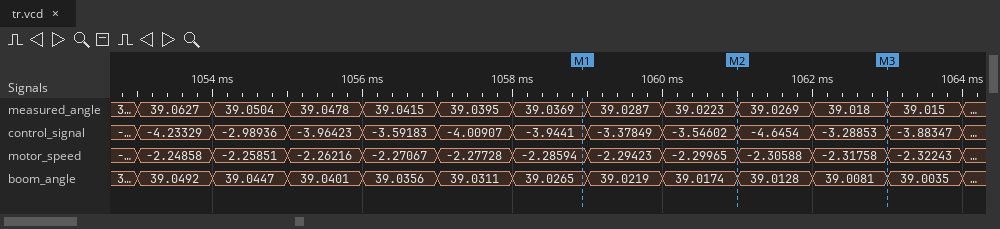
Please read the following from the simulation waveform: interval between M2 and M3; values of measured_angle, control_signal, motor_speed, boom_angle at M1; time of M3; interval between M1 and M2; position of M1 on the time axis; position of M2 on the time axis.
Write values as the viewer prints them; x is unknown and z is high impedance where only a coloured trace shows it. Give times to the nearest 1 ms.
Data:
2 ms
measured_angle=39.0369, control_signal=-3.9441, motor_speed=-2.28594, boom_angle=39.0265
1063 ms
2 ms
1059 ms
1061 ms
